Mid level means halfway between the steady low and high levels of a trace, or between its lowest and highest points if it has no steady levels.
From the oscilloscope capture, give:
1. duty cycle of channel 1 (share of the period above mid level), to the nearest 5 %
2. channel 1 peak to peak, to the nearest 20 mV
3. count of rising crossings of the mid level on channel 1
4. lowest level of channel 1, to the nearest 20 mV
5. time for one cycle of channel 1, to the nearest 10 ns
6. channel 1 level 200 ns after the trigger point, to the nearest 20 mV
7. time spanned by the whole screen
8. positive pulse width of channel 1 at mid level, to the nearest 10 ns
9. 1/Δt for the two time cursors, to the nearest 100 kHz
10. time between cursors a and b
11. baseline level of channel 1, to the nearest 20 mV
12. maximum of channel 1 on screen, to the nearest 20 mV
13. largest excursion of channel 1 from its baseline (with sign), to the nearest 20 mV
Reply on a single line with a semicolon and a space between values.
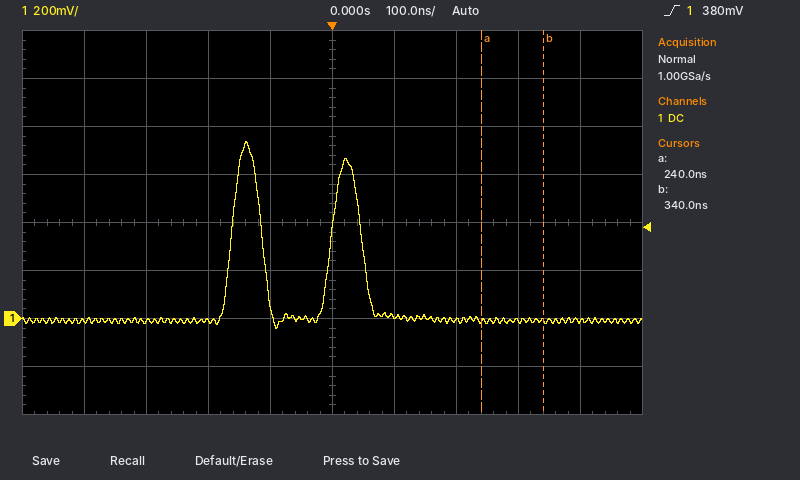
30 %; 780 mV; 2; -40 mV; 160 ns; 0 mV; 1 µs; 50 ns; 10.0 MHz; 100 ns; 0 mV; 740 mV; +740 mV
